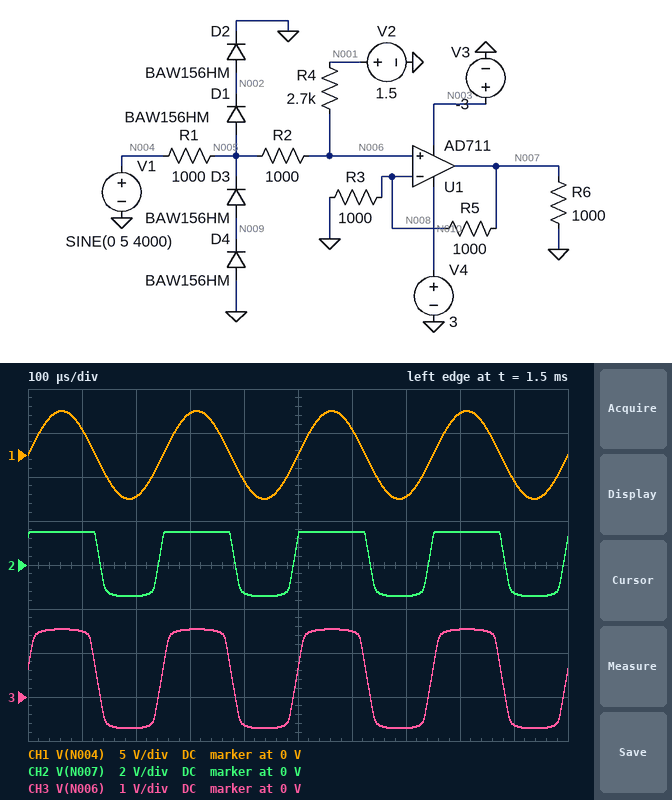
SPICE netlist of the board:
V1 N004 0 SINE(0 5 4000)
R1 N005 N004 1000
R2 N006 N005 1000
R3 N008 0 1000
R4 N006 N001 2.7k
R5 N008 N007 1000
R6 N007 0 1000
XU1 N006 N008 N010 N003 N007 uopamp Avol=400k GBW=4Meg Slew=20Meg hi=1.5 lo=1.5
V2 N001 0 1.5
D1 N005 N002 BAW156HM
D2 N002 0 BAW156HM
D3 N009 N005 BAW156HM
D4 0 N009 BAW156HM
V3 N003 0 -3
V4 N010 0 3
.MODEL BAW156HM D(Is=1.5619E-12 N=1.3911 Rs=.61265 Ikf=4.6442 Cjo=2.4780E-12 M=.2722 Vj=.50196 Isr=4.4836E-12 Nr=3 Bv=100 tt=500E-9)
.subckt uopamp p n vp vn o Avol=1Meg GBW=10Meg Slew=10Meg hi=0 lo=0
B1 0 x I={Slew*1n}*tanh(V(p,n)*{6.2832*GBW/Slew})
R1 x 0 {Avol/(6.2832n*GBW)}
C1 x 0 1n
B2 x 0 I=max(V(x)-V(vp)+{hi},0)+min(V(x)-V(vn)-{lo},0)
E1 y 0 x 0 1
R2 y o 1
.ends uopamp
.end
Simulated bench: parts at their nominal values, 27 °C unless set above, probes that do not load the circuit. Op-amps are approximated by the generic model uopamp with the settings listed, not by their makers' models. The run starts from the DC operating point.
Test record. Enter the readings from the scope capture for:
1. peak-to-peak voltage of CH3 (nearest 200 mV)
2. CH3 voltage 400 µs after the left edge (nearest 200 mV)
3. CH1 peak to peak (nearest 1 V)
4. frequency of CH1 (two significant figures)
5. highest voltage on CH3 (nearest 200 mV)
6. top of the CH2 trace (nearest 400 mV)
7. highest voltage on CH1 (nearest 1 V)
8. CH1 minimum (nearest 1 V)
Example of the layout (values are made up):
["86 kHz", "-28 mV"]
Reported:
["2.2 V", "-600 mV", "10 V", "4.0 kHz", "1.6 V", "1.6 V", "5 V", "-5 V"]
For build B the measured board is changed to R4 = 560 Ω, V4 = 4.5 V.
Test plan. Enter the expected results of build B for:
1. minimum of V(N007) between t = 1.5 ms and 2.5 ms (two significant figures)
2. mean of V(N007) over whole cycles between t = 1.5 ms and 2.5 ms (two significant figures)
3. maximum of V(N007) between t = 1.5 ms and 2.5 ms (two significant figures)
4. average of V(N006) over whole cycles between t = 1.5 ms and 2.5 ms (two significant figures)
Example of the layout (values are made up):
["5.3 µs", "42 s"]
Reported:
["850 mV", "2.1 V", "3.0 V", "1.0 V"]
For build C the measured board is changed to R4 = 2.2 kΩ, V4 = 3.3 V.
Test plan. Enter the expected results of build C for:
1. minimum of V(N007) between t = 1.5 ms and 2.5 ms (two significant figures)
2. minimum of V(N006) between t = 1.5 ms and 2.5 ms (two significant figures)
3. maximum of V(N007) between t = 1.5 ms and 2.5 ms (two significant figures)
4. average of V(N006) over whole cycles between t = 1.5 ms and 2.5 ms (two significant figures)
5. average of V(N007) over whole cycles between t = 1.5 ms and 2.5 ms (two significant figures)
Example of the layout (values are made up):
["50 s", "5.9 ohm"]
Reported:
["-1.2 V", "-580 mV", "1.8 V", "540 mV", "550 mV"]
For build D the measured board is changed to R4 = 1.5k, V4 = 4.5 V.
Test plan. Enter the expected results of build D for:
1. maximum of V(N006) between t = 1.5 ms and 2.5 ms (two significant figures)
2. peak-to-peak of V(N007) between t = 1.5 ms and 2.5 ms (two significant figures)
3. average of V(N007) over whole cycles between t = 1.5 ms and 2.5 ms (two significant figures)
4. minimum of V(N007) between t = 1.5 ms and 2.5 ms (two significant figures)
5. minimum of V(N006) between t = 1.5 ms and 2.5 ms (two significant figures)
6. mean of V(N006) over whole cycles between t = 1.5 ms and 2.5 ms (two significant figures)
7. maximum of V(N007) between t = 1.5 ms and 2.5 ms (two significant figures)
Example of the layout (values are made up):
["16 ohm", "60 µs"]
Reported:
["1.5 V", "3.6 V", "1.3 V", "-630 mV", "-310 mV", "680 mV", "3.0 V"]
